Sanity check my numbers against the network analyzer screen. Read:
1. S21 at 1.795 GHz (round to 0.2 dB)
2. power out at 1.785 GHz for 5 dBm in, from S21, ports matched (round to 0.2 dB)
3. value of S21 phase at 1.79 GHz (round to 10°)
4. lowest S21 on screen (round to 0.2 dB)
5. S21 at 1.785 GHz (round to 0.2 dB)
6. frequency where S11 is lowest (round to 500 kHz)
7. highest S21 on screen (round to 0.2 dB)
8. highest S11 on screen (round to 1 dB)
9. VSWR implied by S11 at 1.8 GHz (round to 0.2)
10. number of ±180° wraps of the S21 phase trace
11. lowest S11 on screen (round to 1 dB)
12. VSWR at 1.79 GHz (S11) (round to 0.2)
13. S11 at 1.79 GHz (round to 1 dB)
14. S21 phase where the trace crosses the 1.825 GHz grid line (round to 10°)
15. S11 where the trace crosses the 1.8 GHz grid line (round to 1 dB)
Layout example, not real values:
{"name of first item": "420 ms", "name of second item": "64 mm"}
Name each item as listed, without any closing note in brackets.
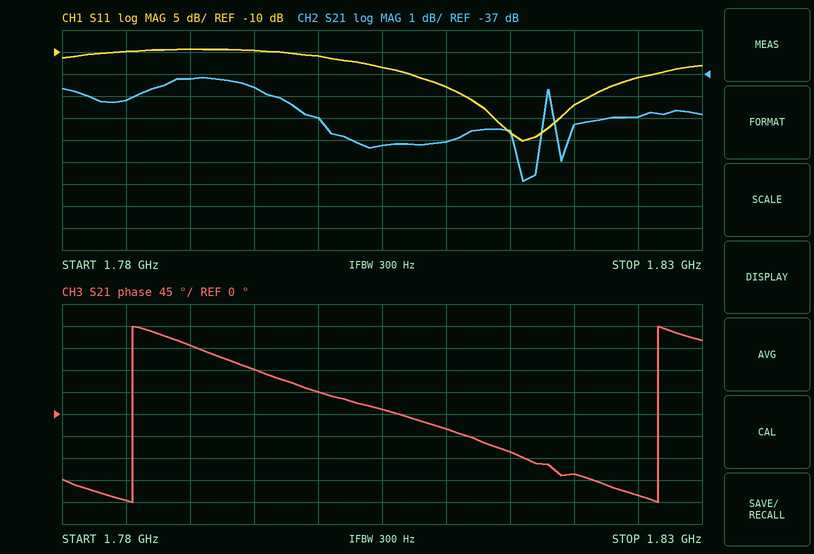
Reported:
{"S21 at 1.795 GHz": "-37.6 dB", "power out at 1.785 GHz for 5 dBm in, from S21, ports matched": "-33.2 dBm", "value of S21 phase at 1.79 GHz": "140°", "lowest S21 on screen": "-41.8 dB", "S21 at 1.785 GHz": "-38.2 dB", "frequency where S11 is lowest": "1.8160 GHz", "highest S21 on screen": "-37.2 dB", "highest S11 on screen": "-9 dB", "VSWR implied by S11 at 1.8 GHz": "1.8", "number of ±180° wraps of the S21 phase trace": "2", "lowest S11 on screen": "-30 dB", "VSWR at 1.79 GHz (S11)": "2.0", "S11 at 1.79 GHz": "-9 dB", "S21 phase where the trace crosses the 1.825 GHz grid line": "-170°", "S11 where the trace crosses the 1.8 GHz grid line": "-11 dB"}
